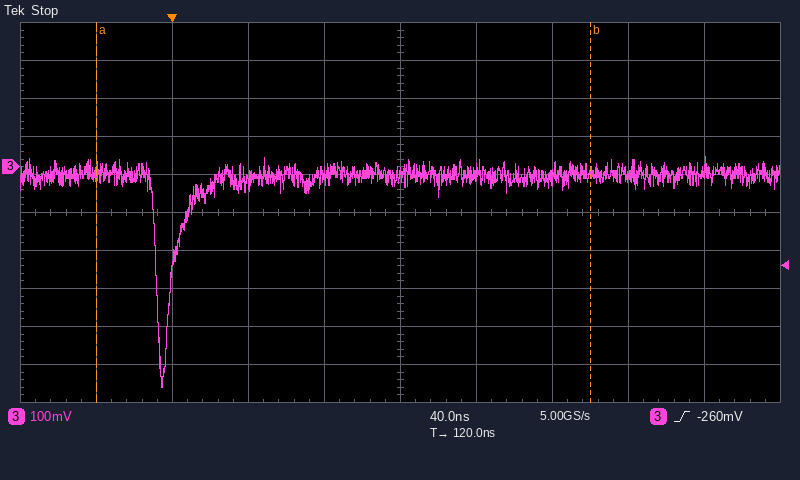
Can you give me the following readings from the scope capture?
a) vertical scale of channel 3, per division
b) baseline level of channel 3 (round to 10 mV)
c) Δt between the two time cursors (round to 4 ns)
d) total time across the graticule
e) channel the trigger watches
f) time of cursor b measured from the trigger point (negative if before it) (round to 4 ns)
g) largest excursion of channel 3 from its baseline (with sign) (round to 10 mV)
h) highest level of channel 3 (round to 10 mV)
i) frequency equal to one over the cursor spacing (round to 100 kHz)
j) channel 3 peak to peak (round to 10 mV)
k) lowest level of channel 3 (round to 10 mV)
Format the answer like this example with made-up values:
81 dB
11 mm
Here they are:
100 mV
-20 mV
260 ns
400 ns
channel 3
+220 ns
-560 mV
30 mV
3.8 MHz
610 mV
-580 mV
